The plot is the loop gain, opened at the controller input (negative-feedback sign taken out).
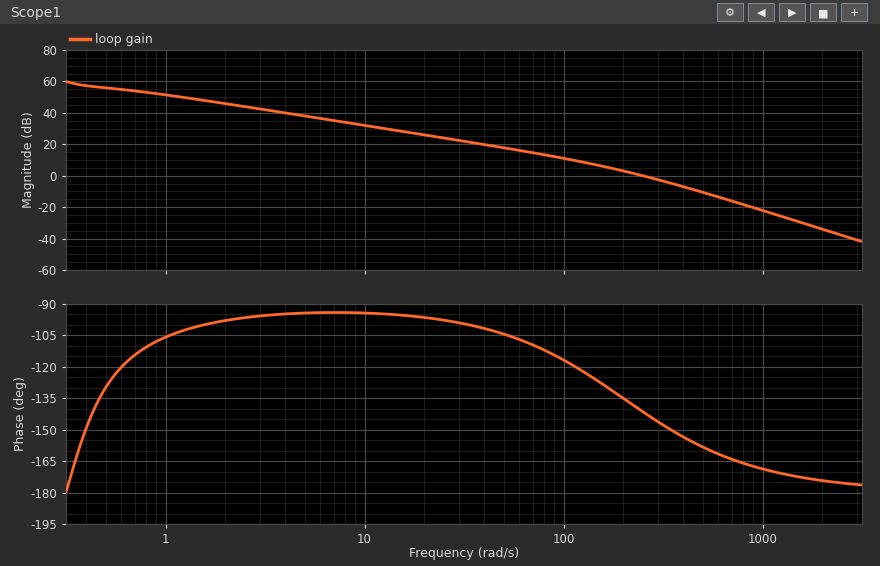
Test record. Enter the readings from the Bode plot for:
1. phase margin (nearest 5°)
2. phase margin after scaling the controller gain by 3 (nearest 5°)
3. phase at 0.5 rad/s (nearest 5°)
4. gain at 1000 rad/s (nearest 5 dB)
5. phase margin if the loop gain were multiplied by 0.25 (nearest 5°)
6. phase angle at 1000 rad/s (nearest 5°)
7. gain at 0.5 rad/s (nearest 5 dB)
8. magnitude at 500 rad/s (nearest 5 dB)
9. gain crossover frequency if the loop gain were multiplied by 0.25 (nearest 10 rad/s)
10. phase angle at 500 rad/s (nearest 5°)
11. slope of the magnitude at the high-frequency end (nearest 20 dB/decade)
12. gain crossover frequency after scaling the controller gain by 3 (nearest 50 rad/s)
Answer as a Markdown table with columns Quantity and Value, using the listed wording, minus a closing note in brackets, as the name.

| Quantity | Value |
|---|---|
| phase margin | 40° |
| phase margin after scaling the controller gain by 3 | 25° |
| phase at 0.5 rad/s | -130° |
| gain at 1000 rad/s | -20 dB |
| phase margin if the loop gain were multiplied by 0.25 | 65° |
| phase angle at 1000 rad/s | -170° |
| gain at 0.5 rad/s | 55 dB |
| magnitude at 500 rad/s | -10 dB |
| gain crossover frequency if the loop gain were multiplied by 0.25 | 90 rad/s |
| phase angle at 500 rad/s | -160° |
| slope of the magnitude at the high-frequency end | -40 dB/decade |
| gain crossover frequency after scaling the controller gain by 3 | 450 rad/s |
